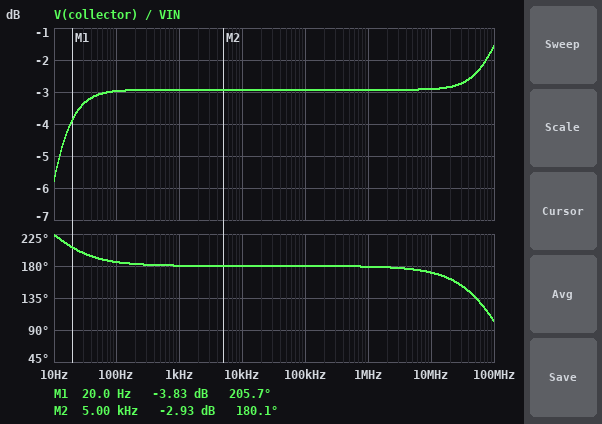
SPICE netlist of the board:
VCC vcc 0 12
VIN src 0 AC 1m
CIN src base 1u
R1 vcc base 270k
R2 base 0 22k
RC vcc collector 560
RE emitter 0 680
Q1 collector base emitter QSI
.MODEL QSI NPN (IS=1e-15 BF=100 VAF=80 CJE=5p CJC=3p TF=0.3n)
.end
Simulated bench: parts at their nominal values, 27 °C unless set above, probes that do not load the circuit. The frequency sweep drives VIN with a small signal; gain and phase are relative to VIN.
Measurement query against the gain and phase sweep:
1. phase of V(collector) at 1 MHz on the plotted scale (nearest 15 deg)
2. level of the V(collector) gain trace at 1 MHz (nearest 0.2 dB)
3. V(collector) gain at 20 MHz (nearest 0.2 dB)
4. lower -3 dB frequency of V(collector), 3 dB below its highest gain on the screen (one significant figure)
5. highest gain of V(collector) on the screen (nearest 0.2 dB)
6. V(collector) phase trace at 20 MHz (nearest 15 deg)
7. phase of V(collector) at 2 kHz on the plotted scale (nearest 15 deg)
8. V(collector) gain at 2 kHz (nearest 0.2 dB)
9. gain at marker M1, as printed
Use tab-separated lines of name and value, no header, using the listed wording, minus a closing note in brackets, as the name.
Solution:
phase of V(collector) at 1 MHz on the plotted scale	180 deg
level of the V(collector) gain trace at 1 MHz	-3.0 dB
V(collector) gain at 20 MHz	-2.8 dB
lower -3 dB frequency of V(collector), 3 dB below its highest gain on the screen	10 Hz
highest gain of V(collector) on the screen	-1.6 dB
V(collector) phase trace at 20 MHz	165 deg
phase of V(collector) at 2 kHz on the plotted scale	180 deg
V(collector) gain at 2 kHz	-3.0 dB
gain at marker M1, as printed	-3.83 dB
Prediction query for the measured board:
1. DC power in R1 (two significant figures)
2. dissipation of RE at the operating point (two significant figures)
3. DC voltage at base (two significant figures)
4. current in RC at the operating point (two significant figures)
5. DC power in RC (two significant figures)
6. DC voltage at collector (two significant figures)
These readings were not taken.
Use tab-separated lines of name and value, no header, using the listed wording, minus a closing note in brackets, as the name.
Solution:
DC power in R1	460 µW
dissipation of RE at the operating point	48 µW
DC voltage at base	860 mV
current in RC at the operating point	260 µA
DC power in RC	39 µW
DC voltage at collector	12 V
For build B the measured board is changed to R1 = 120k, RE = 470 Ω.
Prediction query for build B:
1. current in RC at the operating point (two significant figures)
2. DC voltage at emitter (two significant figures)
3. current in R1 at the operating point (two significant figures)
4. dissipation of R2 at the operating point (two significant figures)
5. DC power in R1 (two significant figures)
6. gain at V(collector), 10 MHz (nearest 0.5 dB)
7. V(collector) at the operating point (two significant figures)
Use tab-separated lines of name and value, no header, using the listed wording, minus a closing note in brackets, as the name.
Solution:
current in RC at the operating point	1.8 mA
DC voltage at emitter	840 mV
current in R1 at the operating point	87 µA
dissipation of R2 at the operating point	110 µW
DC power in R1	910 µW
gain at V(collector), 10 MHz	1.0 dB
V(collector) at the operating point	11 V
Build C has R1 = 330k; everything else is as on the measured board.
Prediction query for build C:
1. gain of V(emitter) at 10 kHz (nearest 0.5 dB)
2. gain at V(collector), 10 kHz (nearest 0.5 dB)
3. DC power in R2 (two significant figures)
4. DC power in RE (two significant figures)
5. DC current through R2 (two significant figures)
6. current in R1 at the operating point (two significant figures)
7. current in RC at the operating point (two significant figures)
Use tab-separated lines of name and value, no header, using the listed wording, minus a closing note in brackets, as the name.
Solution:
gain of V(emitter) at 10 kHz	-2.5 dB
gain at V(collector), 10 kHz	-4.5 dB
DC power in R2	24 µW
DC power in RE	8.4 µW
DC current through R2	33 µA
current in R1 at the operating point	34 µA
current in RC at the operating point	110 µA
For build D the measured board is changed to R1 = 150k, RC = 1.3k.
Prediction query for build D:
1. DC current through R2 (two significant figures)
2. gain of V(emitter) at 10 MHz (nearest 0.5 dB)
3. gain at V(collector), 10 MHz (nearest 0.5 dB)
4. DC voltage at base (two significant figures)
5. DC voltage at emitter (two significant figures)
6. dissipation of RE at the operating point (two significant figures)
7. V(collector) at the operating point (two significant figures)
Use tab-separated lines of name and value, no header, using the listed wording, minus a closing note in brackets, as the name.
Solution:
DC current through R2	62 µA
gain of V(emitter) at 10 MHz	-0.5 dB
gain at V(collector), 10 MHz	5.0 dB
DC voltage at base	1.4 V
DC voltage at emitter	660 mV
dissipation of RE at the operating point	640 µW
V(collector) at the operating point	11 V
